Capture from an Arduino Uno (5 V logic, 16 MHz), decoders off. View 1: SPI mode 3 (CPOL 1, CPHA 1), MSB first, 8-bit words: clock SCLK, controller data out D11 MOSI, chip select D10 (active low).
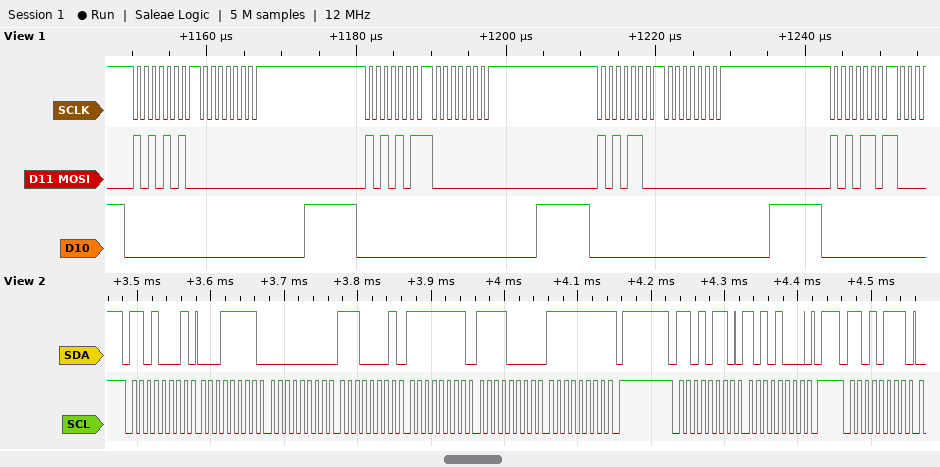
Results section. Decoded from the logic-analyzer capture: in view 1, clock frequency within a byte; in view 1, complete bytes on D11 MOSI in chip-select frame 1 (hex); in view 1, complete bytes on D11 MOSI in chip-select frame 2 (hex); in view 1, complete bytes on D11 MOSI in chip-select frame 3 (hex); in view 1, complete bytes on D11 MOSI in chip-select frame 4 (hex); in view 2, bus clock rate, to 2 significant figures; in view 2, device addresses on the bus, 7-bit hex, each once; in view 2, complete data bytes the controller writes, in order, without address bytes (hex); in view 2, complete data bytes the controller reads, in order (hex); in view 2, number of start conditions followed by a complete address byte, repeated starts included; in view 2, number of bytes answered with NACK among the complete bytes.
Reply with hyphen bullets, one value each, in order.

- 1 MHz
- AA 00
- AB 00
- AC 00
- AD
- 100 kHz
- 0x68 0x6B
- A8
- 1F 00 E1 FF F0 FF
- 3
- 1
